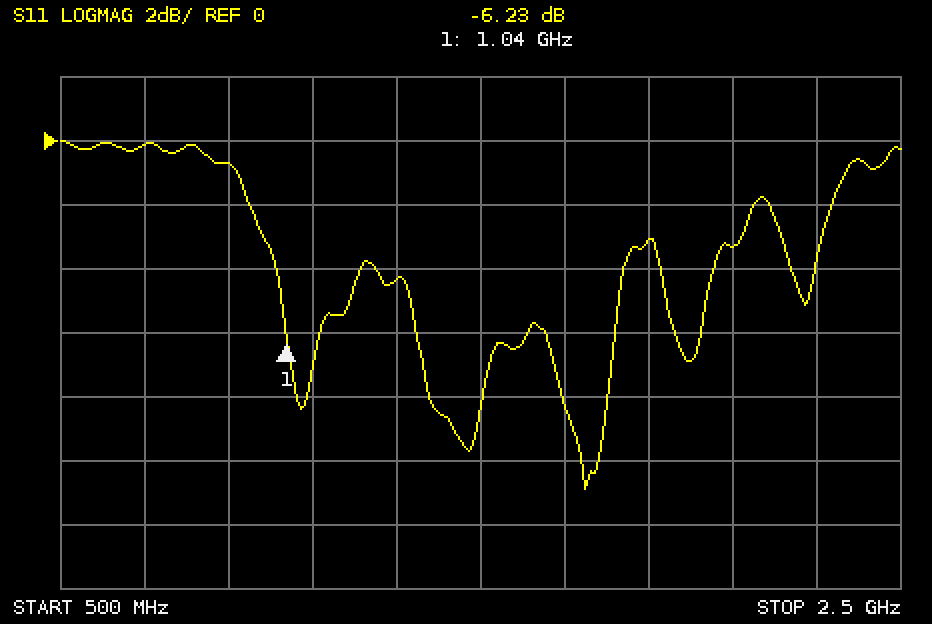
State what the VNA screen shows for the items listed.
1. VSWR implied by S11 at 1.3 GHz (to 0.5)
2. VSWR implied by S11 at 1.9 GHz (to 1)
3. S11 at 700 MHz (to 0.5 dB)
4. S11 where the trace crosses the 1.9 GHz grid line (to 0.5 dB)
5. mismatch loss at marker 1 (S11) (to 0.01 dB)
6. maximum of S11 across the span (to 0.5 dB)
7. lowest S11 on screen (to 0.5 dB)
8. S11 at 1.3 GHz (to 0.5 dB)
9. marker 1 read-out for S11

4.0
6
0.0 dB
-3.0 dB
1.18 dB
0.0 dB
-11.0 dB
-4.5 dB
-6.23 dB
